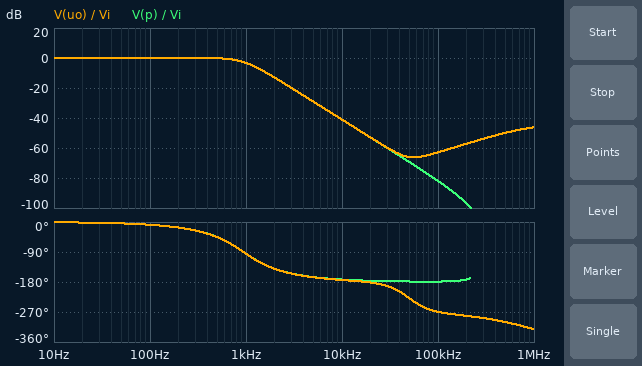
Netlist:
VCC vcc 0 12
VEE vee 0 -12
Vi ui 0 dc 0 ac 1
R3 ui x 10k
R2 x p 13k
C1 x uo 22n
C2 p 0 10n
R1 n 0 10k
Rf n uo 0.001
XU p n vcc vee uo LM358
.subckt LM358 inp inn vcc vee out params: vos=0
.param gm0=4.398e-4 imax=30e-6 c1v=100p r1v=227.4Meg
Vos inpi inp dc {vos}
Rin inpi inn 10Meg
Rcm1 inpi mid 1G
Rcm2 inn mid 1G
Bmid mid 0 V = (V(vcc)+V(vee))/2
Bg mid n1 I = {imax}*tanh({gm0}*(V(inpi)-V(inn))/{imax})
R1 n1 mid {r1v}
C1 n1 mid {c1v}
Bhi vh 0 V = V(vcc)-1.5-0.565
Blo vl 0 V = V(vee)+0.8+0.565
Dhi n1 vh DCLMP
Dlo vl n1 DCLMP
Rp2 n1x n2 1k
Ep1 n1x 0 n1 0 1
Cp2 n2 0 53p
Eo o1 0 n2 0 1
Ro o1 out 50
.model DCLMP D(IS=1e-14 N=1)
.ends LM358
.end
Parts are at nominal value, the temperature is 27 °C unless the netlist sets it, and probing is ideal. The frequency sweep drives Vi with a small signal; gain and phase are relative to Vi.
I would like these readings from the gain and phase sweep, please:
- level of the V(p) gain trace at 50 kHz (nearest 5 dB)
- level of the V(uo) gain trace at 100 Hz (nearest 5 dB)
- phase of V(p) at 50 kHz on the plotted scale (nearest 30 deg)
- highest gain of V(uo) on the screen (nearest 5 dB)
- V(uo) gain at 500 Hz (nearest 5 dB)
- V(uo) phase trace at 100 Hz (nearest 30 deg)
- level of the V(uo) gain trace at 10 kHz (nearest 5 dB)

-70 dB
0 dB
-180 deg
0 dB
0 dB
0 deg
-40 dB
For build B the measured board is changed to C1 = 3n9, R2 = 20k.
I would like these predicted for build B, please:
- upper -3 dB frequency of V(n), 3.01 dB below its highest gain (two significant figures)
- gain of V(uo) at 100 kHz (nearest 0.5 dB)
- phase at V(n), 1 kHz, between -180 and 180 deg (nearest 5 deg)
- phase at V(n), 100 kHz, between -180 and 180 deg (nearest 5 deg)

580 Hz
-62.0 dB
-70 deg
110 deg
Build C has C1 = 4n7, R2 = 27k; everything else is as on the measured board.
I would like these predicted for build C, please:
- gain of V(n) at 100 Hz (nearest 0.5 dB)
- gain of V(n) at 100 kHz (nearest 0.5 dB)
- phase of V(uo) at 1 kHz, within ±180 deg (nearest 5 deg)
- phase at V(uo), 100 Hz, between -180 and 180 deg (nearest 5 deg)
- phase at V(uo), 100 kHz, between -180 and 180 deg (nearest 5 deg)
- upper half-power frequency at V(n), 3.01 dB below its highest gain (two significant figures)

0 dB
-62.5 dB
-80 deg
-15 deg
100 deg
470 Hz
